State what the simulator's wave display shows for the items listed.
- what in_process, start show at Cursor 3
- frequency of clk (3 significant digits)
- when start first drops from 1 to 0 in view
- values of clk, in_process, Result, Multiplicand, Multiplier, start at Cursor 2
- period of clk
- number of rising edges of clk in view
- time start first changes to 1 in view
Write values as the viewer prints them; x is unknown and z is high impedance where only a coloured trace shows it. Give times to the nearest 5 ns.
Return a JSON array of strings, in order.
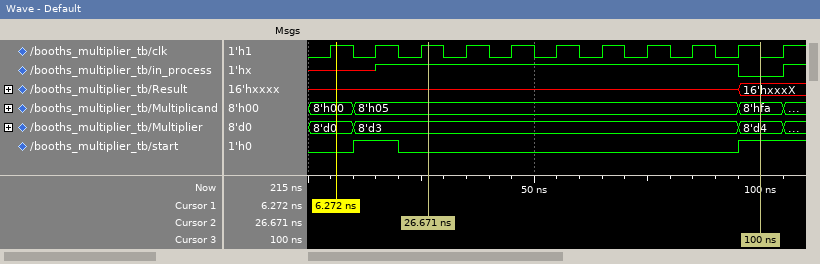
["in_process=0, start=1", "100 MHz", "20 ns", "clk=1, in_process=1, Result=x, Multiplicand=8'h05, Multiplier=8'd3, start=0", "10 ns", "11", "10 ns"]
